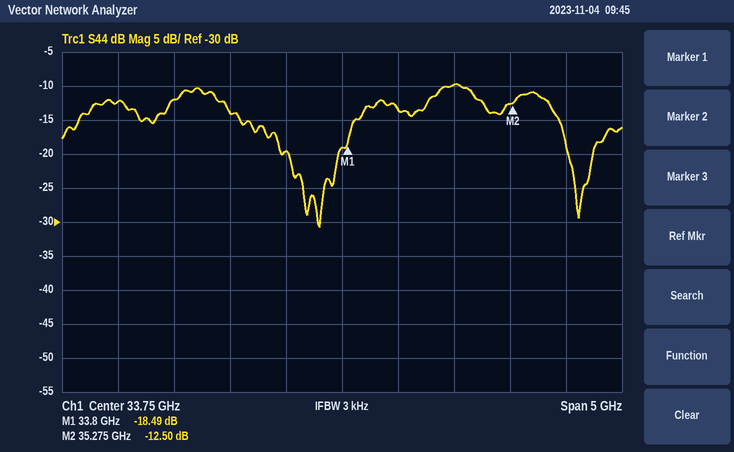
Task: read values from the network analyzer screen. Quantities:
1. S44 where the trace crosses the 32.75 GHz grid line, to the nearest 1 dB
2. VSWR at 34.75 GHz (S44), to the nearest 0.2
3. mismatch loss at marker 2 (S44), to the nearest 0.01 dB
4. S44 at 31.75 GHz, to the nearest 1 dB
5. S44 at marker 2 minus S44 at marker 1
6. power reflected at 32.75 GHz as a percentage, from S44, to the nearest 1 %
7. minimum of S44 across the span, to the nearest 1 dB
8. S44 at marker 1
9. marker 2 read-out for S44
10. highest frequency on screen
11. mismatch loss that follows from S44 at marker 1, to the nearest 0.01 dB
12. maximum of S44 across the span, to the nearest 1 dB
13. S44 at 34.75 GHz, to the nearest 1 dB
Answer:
-14 dB
2.0
0.25 dB
-12 dB
5.99 dB
4 %
-31 dB
-18.49 dB
-12.50 dB
36.25 GHz
0.06 dB
-10 dB
-10 dB
